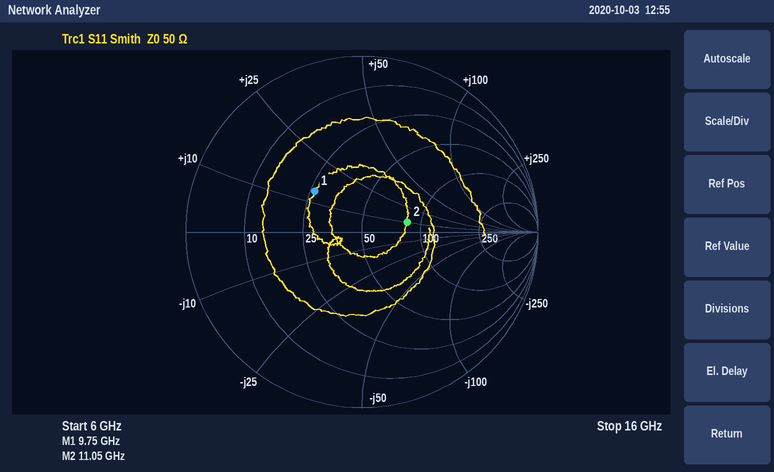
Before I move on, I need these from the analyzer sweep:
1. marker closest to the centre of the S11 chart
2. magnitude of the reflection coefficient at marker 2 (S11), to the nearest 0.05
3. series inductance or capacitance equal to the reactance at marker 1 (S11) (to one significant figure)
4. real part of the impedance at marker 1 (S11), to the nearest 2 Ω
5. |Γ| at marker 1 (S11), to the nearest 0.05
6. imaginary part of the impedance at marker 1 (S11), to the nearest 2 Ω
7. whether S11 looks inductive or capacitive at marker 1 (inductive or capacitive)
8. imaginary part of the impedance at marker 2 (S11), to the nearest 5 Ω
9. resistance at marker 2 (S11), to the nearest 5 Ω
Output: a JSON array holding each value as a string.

["marker 2", "0.25", "200 pH", "26 Ω", "0.35", "+14 Ω", "inductive", "+10 Ω", "85 Ω"]
